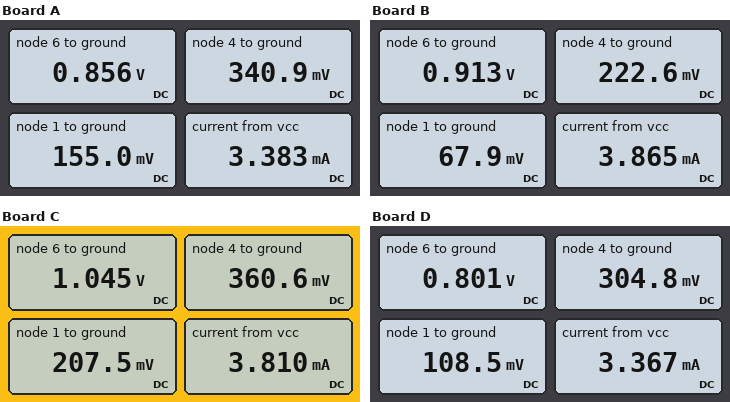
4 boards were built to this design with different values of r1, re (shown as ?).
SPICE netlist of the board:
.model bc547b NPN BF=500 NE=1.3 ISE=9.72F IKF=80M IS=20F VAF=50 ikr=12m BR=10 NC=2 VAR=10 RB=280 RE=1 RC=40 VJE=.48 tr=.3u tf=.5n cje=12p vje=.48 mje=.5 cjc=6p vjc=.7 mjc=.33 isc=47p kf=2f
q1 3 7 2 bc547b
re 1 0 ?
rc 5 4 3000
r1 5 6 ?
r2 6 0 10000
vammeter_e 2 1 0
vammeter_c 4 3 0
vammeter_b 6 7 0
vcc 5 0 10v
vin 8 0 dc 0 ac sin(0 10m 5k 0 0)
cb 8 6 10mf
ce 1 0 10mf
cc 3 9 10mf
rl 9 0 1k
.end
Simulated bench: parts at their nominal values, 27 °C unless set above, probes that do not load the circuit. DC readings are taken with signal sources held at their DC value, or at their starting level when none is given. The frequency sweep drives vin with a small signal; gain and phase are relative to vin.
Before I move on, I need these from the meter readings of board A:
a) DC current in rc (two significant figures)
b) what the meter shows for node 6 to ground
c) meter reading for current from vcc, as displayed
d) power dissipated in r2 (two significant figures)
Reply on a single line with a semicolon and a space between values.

3.2 mA; 0.856 V; 3.383 mA; 73 µW
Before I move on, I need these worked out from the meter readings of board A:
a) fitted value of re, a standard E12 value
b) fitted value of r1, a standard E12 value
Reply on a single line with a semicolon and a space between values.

47 Ω; 56 kΩ
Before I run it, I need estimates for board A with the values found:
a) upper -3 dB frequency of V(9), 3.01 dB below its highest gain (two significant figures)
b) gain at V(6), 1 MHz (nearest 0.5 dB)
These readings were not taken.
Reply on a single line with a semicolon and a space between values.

73 kHz; 0 dB
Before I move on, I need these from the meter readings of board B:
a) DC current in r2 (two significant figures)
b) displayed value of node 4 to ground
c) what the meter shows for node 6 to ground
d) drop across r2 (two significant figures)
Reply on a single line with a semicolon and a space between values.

91 µA; 222.6 mV; 0.913 V; 910 mV
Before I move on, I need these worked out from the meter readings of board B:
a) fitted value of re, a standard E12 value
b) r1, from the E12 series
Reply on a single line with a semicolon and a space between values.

18 Ω; 15 kΩ
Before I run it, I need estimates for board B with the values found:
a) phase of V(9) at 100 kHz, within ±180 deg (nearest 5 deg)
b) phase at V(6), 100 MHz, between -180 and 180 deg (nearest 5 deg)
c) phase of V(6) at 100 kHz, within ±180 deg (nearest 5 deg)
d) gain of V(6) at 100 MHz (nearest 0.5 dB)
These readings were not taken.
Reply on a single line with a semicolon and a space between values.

95 deg; 0 deg; 0 deg; 0 dB
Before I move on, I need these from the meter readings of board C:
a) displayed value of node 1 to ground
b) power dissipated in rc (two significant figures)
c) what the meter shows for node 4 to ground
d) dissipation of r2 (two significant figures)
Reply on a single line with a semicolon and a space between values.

207.5 mV; 31 mW; 360.6 mV; 110 µW
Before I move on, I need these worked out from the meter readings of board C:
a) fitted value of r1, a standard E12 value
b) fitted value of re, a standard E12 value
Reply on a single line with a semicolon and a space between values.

15 kΩ; 56 Ω
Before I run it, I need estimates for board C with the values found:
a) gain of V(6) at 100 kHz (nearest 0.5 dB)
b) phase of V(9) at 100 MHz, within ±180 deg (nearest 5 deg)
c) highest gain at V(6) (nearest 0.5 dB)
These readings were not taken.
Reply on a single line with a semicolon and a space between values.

0 dB; -15 deg; 0 dB
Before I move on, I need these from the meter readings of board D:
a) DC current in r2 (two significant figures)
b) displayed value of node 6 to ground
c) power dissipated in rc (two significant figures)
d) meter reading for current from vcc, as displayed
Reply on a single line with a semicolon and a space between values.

80 µA; 0.801 V; 31 mW; 3.367 mA
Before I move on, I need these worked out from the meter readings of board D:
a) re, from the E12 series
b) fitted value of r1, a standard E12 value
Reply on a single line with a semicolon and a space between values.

33 Ω; 68 kΩ
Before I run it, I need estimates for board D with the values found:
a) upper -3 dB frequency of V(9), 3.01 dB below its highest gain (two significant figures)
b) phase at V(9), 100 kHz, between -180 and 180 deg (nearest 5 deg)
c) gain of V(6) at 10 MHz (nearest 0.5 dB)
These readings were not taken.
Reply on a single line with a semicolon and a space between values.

76 kHz; 125 deg; 0 dB
